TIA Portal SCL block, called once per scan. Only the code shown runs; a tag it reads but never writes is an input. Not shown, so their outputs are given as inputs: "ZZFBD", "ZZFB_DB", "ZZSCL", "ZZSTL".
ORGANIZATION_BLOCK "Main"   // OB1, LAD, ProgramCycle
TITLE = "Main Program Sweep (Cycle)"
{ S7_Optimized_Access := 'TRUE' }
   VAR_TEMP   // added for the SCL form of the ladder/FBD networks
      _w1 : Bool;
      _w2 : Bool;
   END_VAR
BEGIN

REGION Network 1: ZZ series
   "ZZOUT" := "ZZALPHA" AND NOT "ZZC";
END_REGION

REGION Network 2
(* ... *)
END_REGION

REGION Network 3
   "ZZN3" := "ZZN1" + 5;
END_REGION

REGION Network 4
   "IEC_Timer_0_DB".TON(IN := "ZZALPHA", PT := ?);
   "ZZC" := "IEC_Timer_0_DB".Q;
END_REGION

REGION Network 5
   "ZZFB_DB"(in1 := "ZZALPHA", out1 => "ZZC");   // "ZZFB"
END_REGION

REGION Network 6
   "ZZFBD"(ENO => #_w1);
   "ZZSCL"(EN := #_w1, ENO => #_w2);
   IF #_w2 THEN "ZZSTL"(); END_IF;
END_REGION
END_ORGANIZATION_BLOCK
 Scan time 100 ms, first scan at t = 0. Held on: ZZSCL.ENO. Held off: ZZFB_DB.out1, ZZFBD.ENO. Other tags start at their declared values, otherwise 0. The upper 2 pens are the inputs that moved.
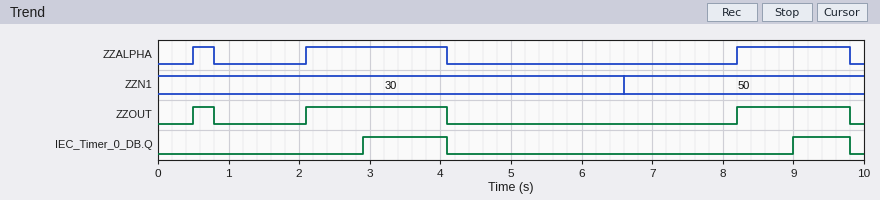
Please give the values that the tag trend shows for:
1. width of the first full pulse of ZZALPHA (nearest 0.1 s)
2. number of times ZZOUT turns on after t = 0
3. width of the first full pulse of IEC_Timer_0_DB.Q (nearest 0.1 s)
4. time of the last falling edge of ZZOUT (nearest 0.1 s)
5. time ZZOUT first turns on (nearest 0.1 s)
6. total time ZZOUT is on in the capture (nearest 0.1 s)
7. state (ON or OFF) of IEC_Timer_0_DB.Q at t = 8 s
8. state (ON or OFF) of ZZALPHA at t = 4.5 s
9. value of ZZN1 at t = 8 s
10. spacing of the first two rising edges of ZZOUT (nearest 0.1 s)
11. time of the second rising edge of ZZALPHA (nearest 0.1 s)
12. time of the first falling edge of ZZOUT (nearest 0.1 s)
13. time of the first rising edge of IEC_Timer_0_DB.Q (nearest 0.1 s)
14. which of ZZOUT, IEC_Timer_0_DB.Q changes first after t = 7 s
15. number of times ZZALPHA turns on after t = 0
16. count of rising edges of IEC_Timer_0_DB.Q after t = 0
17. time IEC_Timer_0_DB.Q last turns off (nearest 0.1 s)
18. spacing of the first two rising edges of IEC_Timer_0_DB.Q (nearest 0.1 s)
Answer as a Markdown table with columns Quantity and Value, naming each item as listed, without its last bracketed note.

| Quantity | Value |
|---|---|
| width of the first full pulse of ZZALPHA | 0.3 s |
| number of times ZZOUT turns on after t = 0 | 3 |
| width of the first full pulse of IEC_Timer_0_DB.Q | 1.2 s |
| time of the last falling edge of ZZOUT | 9.8 s |
| time ZZOUT first turns on | 0.5 s |
| total time ZZOUT is on in the capture | 3.9 s |
| state (ON or OFF) of IEC_Timer_0_DB.Q at t = 8 s | OFF |
| state (ON or OFF) of ZZALPHA at t = 4.5 s | OFF |
| value of ZZN1 at t = 8 s | 50 |
| spacing of the first two rising edges of ZZOUT | 1.6 s |
| time of the second rising edge of ZZALPHA | 2.1 s |
| time of the first falling edge of ZZOUT | 0.8 s |
| time of the first rising edge of IEC_Timer_0_DB.Q | 2.9 s |
| which of ZZOUT, IEC_Timer_0_DB.Q changes first after t = 7 s | ZZOUT |
| number of times ZZALPHA turns on after t = 0 | 3 |
| count of rising edges of IEC_Timer_0_DB.Q after t = 0 | 2 |
| time IEC_Timer_0_DB.Q last turns off | 9.8 s |
| spacing of the first two rising edges of IEC_Timer_0_DB.Q | 6.1 s |
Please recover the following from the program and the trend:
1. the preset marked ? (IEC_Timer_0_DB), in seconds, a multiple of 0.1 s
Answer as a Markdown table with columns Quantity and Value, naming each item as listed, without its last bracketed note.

| Quantity | Value |
|---|---|
| the preset marked ? (IEC_Timer_0_DB), in seconds, a multiple of 0.1 s | 0.8 s |
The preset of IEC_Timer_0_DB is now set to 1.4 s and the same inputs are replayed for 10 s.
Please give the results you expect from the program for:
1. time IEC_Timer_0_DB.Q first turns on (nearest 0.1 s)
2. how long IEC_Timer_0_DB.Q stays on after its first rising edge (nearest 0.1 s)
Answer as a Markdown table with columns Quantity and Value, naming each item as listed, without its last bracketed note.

| Quantity | Value |
|---|---|
| time IEC_Timer_0_DB.Q first turns on | 3.5 s |
| how long IEC_Timer_0_DB.Q stays on after its first rising edge | 0.6 s |
